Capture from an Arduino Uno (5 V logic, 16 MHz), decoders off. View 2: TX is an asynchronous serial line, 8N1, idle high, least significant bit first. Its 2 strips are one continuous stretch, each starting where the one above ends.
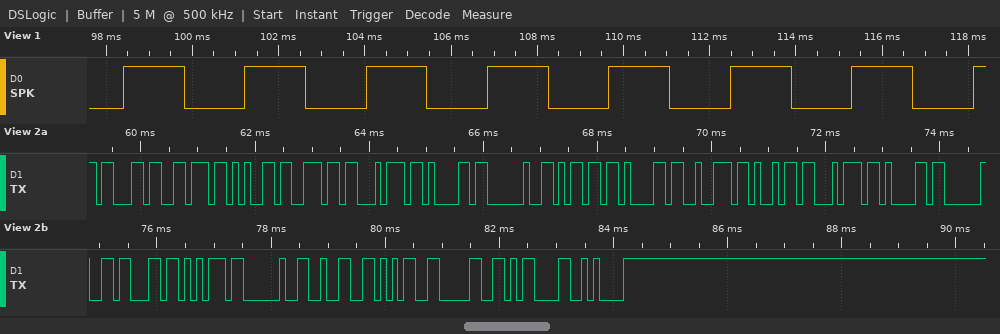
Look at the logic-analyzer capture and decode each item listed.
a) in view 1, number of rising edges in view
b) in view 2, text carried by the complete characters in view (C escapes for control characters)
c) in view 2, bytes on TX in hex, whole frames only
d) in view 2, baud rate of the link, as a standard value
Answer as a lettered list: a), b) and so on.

a) 8
b) "cventa marita cu 250\r\n"
c) 0x63 0x76 0x65 0x6E 0x74 0x61 0x20 0x6D 0x61 0x72 0x69 0x74 0x61 0x20 0x63 0x75 0x20 0x32 0x35 0x30 0x0D 0x0A
d) 9600 baud
